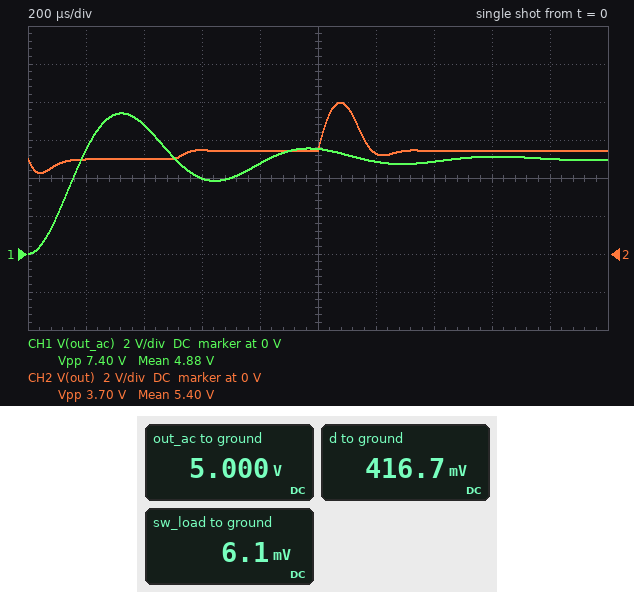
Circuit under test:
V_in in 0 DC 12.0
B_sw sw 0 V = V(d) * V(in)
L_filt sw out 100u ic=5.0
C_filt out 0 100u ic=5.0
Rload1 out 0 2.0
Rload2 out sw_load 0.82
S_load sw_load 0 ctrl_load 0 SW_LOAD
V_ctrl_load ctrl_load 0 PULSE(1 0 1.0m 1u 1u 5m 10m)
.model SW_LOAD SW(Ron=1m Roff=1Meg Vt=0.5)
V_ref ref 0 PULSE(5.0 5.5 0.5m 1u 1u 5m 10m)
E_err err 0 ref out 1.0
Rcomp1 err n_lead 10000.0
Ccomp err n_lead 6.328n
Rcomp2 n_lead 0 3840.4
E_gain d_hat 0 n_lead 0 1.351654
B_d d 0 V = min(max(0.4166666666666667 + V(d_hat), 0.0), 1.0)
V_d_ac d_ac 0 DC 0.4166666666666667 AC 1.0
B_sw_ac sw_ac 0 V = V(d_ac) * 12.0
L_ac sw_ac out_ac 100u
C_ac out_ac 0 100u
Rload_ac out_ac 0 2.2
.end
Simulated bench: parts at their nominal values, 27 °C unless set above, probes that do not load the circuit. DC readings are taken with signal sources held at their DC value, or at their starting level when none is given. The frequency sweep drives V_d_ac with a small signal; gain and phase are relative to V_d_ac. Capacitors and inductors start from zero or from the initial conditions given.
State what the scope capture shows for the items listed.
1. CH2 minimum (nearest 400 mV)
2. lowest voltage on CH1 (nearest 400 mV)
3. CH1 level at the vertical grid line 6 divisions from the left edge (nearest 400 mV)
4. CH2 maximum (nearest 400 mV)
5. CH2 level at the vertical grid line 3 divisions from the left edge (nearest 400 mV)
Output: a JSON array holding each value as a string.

["4.4 V", "0 V", "4.8 V", "8.0 V", "5.6 V"]
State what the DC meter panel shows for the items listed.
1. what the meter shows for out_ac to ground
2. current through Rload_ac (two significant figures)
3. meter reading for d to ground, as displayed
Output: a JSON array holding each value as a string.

["5.000 V", "2.3 A", "416.7 mV"]
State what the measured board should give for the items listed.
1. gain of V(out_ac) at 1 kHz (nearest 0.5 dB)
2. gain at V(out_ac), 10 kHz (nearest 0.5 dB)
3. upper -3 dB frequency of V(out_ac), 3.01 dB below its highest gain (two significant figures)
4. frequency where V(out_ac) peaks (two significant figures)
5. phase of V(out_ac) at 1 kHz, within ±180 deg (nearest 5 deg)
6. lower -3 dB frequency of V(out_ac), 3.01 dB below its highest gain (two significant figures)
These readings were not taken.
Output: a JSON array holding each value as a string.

["25.0 dB", "-10.0 dB", "1.8 kHz", "1.5 kHz", "-25 deg", "1.1 kHz"]
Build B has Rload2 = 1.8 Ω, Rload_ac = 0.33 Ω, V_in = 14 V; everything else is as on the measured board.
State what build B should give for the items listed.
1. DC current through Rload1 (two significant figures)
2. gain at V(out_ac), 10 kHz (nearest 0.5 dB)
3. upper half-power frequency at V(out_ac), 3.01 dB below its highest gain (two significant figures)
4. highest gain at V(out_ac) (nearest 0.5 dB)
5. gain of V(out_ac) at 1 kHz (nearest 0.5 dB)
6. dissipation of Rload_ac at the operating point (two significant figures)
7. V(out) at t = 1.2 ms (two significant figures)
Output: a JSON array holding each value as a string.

["2.6 A", "-11.0 dB", "590 Hz", "21.5 dB", "15.5 dB", "76 W", "5.5 V"]
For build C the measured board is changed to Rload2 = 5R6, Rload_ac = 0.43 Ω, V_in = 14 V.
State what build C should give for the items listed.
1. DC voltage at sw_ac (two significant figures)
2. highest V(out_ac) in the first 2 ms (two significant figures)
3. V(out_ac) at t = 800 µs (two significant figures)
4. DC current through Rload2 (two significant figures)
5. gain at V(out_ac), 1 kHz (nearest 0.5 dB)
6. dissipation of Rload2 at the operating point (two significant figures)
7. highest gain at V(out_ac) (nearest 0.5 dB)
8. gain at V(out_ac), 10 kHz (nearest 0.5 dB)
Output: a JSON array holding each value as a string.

["5.0 V", "5.0 V", "4.9 V", "920 mA", "17.5 dB", "4.7 W", "21.5 dB", "-10.5 dB"]
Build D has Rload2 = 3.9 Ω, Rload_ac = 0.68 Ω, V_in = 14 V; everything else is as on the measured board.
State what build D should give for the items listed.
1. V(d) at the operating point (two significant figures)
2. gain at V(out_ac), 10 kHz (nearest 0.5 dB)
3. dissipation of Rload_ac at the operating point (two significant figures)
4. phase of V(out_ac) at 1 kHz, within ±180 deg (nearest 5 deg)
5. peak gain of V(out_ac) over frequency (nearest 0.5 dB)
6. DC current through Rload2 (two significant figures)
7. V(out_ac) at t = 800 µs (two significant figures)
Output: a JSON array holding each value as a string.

["370 mV", "-10.5 dB", "37 W", "-55 deg", "21.5 dB", "1.3 A", "5.0 V"]
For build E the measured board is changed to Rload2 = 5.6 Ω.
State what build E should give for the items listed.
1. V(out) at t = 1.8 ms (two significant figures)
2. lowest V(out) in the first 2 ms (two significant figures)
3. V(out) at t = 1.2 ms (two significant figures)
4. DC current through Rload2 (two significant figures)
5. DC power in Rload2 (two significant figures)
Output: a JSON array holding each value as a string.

["5.4 V", "5.0 V", "5.4 V", "890 mA", "4.5 W"]
